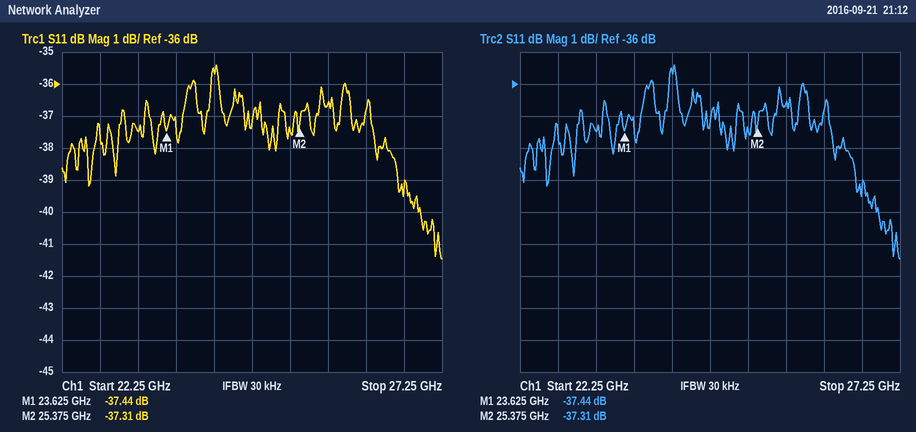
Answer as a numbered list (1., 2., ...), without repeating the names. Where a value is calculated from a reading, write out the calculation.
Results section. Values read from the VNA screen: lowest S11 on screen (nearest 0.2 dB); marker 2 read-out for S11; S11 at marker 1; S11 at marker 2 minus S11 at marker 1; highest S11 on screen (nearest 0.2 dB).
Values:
1. -41.4 dB
2. -37.31 dB
3. -37.44 dB
4. -37.31 − (-37.44) = 0.13 dB
5. -35.4 dB
